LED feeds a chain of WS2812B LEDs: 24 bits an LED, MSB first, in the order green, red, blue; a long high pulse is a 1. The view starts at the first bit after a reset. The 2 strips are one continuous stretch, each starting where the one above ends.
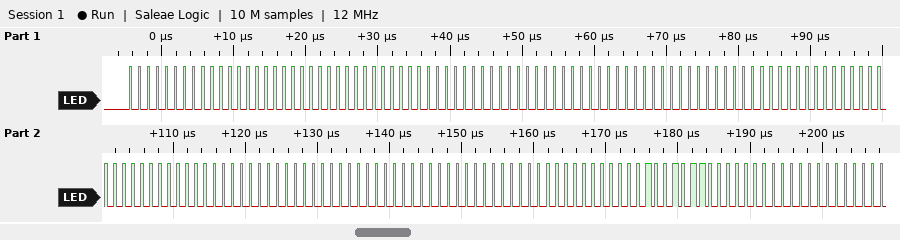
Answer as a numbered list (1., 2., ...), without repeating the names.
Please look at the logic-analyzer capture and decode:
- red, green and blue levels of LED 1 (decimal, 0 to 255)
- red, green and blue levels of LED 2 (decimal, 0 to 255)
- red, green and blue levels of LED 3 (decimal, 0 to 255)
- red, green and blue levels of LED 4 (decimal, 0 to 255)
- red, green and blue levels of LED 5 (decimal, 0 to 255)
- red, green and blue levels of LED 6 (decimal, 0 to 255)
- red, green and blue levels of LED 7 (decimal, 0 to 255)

1. 0, 0, 0
2. 0, 0, 0
3. 0, 0, 0
4. 0, 0, 0
5. 0, 0, 0
6. 0, 0, 0
7. 0, 150, 0
